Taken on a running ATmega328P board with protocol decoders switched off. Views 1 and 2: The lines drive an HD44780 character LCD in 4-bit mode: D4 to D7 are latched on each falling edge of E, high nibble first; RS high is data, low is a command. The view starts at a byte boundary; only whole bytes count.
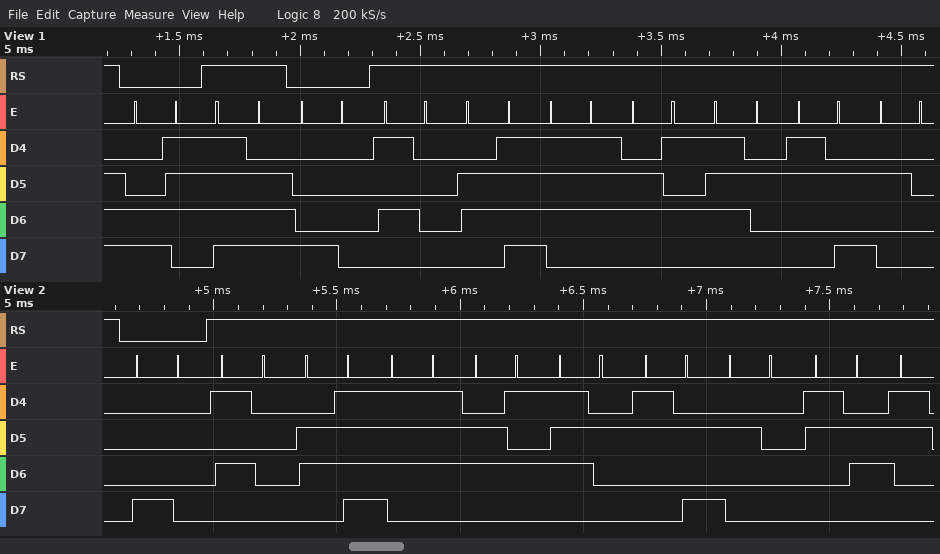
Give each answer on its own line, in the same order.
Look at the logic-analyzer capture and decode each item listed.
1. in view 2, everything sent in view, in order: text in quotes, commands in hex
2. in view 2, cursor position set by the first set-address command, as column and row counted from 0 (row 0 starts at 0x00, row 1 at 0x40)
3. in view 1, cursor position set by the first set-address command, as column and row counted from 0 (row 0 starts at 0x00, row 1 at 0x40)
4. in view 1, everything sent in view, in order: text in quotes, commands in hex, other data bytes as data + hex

0x80 "Power: 6"
column 0, row 0
column 7, row 1
0xC7 data FE 0x80 "Power: "
